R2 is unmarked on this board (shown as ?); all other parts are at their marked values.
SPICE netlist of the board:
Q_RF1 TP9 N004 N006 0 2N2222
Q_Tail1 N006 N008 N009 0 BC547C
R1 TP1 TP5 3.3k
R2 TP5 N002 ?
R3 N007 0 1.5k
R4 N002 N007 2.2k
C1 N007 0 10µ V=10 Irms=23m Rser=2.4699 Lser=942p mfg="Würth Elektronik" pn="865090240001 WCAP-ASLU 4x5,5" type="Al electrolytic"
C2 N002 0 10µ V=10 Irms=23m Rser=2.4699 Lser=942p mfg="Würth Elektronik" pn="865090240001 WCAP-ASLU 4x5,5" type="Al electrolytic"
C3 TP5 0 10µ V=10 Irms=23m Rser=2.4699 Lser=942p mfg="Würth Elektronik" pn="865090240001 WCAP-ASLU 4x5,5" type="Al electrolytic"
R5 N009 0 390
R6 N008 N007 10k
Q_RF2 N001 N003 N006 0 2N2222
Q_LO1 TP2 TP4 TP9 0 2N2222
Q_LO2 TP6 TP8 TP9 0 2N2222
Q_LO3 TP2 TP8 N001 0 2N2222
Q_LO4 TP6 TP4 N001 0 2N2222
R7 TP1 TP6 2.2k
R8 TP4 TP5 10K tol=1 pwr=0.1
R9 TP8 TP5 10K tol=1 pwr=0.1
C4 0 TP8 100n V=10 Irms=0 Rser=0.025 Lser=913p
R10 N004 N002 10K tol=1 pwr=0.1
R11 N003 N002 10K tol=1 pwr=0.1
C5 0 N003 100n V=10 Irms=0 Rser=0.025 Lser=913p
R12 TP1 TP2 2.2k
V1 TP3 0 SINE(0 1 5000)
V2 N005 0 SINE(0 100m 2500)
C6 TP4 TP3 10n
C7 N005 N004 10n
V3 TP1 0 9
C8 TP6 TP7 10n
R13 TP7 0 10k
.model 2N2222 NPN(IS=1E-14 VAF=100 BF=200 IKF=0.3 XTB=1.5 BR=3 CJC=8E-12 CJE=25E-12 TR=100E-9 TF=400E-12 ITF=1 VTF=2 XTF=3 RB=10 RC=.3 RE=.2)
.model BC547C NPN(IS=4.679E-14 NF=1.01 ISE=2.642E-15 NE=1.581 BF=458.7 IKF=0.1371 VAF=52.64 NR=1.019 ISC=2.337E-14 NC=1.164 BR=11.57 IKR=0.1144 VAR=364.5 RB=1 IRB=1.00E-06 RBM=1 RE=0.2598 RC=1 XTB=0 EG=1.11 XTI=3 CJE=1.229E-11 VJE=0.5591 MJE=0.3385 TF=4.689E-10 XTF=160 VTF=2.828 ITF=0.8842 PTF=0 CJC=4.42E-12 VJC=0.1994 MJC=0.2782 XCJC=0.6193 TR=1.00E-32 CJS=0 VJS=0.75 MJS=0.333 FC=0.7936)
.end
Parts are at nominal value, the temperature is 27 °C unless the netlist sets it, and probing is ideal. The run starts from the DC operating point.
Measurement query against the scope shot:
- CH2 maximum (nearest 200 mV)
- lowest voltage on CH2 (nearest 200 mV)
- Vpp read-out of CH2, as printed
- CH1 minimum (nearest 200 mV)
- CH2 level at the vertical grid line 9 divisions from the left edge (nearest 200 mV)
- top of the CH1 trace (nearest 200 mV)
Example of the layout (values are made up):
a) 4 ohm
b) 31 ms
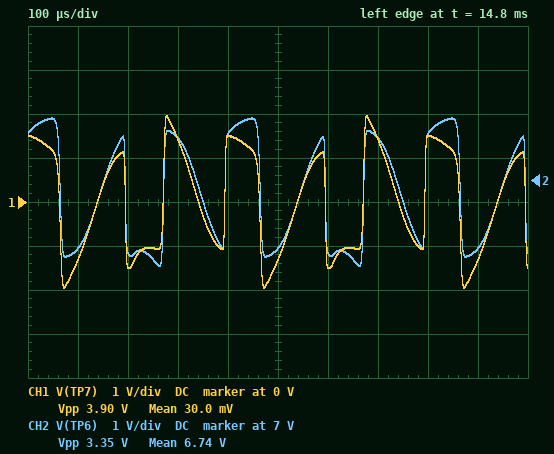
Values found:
a) 8.4 V
b) 5.0 V
c) 3.35 V
d) -2.0 V
e) 5.4 V
f) 2.0 V
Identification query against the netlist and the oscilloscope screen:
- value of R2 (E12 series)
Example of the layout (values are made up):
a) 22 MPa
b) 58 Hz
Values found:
a) 1.8 kΩ
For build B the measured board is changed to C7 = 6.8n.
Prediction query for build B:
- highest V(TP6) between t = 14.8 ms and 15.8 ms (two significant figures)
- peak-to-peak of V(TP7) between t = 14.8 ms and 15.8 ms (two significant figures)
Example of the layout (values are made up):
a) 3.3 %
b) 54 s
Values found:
a) 8.1 V
b) 3.1 V
